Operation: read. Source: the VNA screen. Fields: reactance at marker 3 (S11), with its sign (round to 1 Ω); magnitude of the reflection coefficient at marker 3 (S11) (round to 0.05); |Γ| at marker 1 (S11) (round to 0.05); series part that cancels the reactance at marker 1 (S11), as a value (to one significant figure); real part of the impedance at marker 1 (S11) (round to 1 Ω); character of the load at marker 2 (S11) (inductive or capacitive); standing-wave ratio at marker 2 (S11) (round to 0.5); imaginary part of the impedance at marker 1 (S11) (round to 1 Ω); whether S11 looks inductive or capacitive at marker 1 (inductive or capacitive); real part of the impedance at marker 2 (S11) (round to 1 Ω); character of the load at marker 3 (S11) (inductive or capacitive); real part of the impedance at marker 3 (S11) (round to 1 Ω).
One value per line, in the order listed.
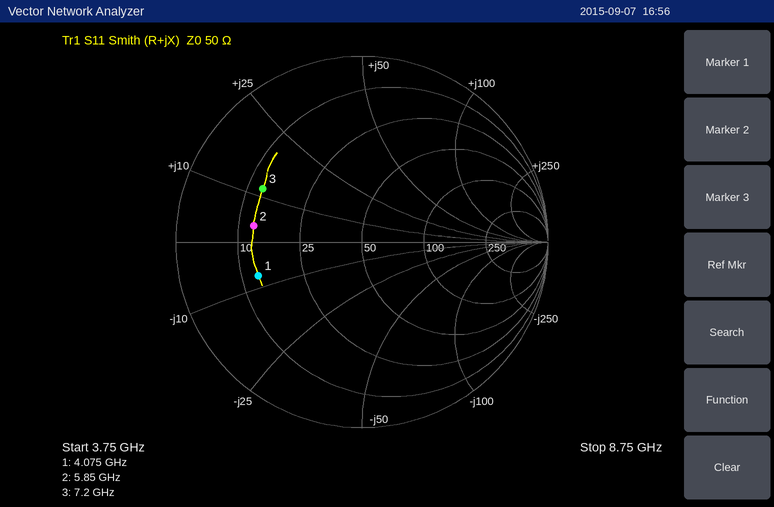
+12 Ω
0.60
0.60
300 pH
13 Ω
inductive
4.0
-7 Ω
capacitive
13 Ω
inductive
13 Ω
